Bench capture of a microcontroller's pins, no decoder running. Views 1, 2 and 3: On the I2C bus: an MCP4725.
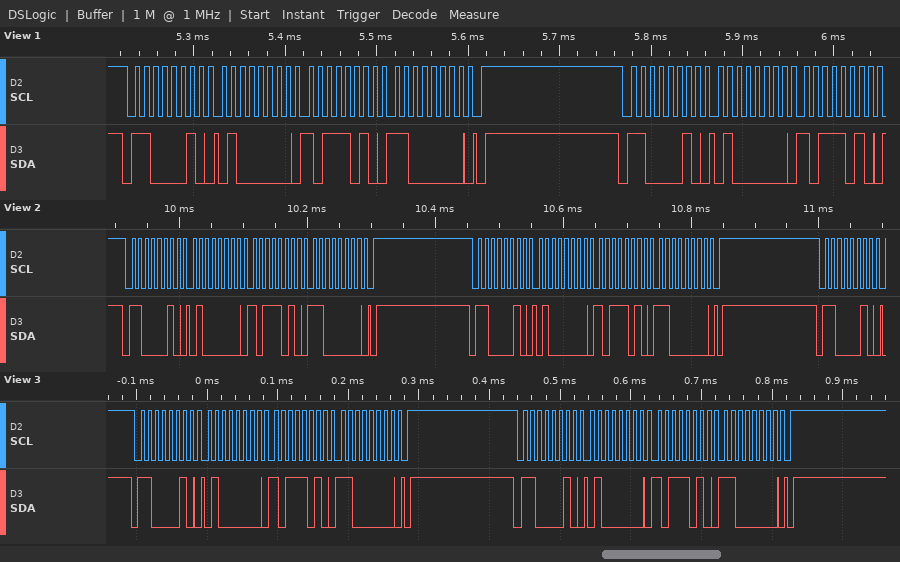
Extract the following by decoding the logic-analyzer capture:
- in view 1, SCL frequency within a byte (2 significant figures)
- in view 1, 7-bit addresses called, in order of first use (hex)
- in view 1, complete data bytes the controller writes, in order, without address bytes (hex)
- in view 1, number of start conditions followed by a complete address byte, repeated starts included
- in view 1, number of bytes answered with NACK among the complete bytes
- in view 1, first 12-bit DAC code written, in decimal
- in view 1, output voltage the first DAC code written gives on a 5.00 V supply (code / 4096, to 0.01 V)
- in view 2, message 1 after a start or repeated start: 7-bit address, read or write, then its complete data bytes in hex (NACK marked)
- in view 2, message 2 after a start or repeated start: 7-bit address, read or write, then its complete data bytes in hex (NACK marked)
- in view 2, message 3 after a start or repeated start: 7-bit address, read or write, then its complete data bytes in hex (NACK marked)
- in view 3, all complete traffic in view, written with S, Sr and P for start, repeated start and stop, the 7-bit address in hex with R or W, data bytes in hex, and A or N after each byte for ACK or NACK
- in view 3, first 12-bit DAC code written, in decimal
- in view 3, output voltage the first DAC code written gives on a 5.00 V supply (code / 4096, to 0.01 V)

100 kHz
0x61
40 BA C0 40 BA
2
0
2988
3.65 V
0x61 write: 40 BA C0
0x61 write: 40 BA C0
0x61 write
S 61W A 40 A BA A C0 A P S 61W A 40 A BA A C0 A P
2988
3.65 V
